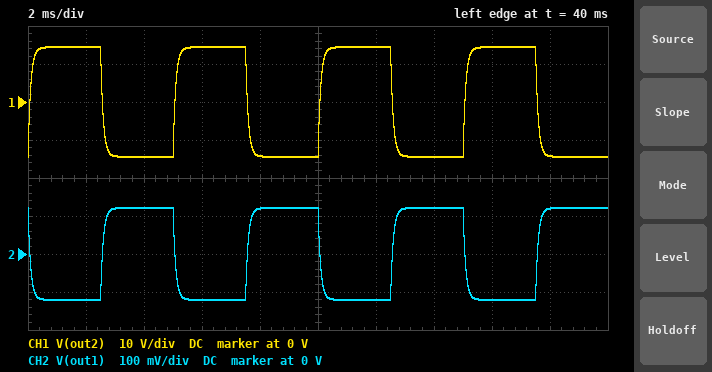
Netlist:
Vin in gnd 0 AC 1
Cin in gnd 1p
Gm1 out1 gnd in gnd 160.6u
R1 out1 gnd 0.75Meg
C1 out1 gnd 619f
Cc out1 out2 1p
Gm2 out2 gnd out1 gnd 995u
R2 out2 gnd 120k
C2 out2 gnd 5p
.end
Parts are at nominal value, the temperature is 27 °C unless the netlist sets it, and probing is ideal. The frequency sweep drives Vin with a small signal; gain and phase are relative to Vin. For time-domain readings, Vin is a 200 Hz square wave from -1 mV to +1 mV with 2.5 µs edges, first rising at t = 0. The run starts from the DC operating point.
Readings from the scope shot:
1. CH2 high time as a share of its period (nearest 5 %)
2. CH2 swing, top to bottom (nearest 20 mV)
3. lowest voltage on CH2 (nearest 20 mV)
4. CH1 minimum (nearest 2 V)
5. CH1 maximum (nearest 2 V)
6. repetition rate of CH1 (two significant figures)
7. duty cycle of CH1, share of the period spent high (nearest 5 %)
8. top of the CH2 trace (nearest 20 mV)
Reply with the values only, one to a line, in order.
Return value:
50 %
240 mV
-120 mV
-14 V
14 V
200 Hz
50 %
120 mV
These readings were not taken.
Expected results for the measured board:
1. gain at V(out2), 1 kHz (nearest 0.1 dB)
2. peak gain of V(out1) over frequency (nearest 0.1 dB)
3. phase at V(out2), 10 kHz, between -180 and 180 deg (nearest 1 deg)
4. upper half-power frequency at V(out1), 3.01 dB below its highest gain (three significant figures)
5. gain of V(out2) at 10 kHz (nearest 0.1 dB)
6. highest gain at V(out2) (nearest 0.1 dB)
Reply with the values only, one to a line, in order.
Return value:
81.9 dB
41.6 dB
-80 deg
1.74 kHz
67.8 dB
83.2 dB
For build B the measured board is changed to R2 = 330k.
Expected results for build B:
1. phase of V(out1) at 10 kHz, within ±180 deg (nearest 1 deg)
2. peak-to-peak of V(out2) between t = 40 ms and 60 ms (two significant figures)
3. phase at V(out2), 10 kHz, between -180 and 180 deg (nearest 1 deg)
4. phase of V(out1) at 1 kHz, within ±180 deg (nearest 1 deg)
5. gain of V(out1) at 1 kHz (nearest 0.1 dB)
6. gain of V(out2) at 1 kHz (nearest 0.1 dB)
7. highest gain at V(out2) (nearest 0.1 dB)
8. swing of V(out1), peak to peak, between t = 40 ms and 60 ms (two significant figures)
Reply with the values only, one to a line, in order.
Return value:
101 deg
79 V
-86 deg
123 deg
36.2 dB
86.6 dB
91.9 dB
240 mV
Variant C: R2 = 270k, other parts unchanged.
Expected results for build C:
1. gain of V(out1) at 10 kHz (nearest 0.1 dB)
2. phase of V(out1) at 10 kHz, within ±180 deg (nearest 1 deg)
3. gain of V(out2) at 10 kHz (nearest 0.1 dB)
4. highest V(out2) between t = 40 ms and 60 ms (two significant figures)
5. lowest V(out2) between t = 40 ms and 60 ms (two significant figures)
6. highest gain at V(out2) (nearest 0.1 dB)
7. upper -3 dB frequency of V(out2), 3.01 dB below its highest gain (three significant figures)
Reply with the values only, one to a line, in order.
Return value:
19.5 dB
100 deg
68.0 dB
32 V
-32 V
90.2 dB
779 Hz
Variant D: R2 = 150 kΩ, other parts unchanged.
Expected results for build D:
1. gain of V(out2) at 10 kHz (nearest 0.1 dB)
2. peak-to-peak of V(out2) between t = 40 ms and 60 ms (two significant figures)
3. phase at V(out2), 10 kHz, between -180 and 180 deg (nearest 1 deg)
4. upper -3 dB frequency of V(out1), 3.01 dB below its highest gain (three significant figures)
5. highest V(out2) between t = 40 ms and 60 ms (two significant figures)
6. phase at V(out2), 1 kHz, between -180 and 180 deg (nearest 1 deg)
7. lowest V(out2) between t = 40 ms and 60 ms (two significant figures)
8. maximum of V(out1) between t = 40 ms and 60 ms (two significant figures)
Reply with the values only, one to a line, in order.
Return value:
67.9 dB
36 V
-82 deg
1.40 kHz
18 V
-36 deg
-18 V
120 mV
